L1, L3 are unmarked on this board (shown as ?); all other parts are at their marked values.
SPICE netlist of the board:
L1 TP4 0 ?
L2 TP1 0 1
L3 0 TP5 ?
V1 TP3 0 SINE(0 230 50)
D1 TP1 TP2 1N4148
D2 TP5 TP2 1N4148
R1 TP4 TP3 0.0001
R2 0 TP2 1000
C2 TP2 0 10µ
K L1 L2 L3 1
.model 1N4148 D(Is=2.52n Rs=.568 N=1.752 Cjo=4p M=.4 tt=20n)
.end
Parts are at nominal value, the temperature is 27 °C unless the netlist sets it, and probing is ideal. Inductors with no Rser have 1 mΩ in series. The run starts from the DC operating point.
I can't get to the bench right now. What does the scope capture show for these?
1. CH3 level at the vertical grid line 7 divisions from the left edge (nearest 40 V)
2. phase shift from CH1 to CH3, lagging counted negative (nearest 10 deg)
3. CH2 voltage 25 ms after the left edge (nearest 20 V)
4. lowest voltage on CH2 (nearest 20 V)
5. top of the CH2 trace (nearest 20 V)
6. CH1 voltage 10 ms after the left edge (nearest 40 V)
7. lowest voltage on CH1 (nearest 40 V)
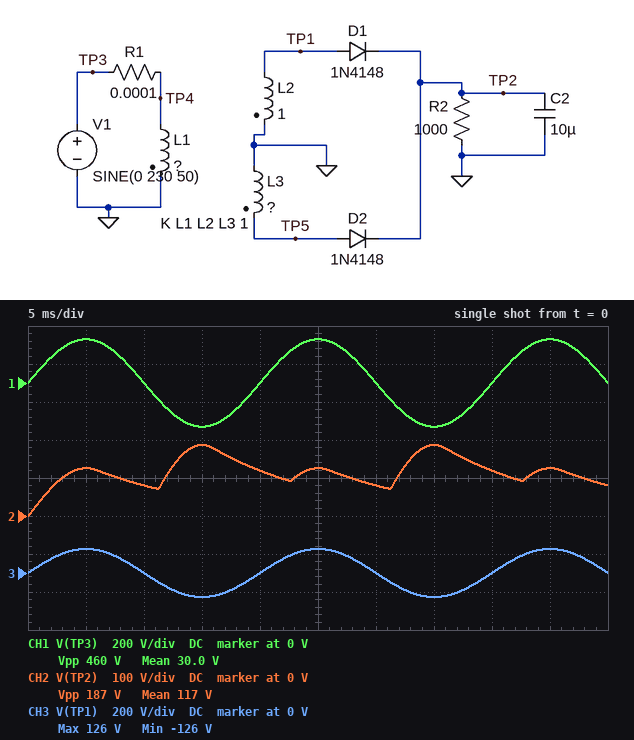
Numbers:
-120 V
0 deg
120 V
0 V
180 V
0 V
-240 V
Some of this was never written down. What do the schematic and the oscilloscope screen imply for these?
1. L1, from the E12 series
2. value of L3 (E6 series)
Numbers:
3.3 H
2.2 H
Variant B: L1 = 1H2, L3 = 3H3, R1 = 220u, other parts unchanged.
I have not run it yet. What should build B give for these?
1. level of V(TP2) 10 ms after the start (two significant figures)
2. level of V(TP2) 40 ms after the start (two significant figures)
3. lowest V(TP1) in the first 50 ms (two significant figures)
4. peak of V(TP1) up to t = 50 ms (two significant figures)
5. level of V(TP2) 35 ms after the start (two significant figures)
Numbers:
130 V
240 V
-210 V
210 V
380 V
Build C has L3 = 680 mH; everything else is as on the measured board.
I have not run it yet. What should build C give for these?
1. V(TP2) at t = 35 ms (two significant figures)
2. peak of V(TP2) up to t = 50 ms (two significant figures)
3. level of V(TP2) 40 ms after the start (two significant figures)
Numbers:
100 V
130 V
66 V
